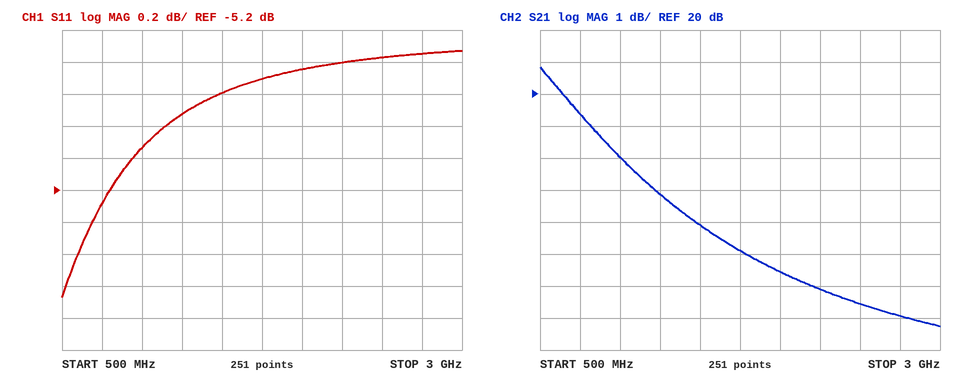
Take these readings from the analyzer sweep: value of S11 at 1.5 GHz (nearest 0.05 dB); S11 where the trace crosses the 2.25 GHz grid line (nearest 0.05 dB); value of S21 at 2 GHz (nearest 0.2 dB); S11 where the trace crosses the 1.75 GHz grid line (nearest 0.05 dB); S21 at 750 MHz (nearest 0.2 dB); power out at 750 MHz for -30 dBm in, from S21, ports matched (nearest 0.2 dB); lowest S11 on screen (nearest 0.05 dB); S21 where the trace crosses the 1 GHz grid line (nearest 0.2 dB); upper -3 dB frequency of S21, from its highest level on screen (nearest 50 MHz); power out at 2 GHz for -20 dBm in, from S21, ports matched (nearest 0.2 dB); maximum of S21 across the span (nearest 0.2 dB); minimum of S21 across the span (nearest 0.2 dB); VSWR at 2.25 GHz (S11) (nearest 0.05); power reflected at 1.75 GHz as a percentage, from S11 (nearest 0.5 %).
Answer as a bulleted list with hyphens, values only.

- -4.60 dB
- -4.40 dB
- 14.4 dB
- -4.50 dB
- 19.4 dB
- -10.6 dBm
- -5.85 dB
- 18.0 dB
- 1.05 GHz
- -5.6 dBm
- 20.8 dB
- 12.8 dB
- 4.05
- 35.5 %
